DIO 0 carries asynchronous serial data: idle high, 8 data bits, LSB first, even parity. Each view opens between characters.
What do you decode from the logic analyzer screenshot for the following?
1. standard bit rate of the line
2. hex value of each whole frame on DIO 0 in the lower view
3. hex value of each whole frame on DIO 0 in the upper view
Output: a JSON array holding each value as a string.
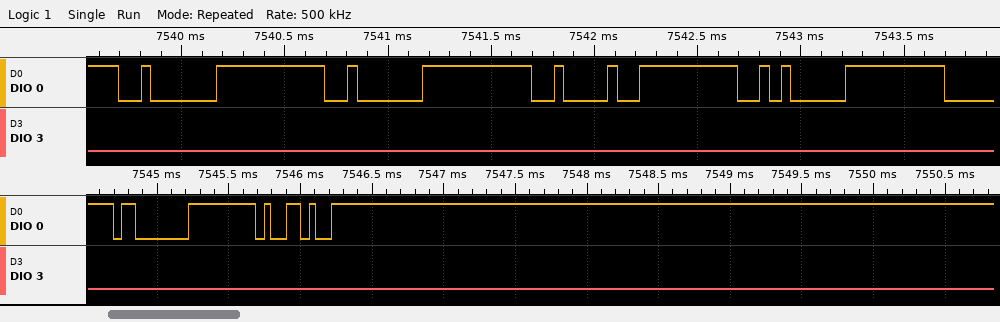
["19200 baud", "03, 59", "02, 02, 42, 0A"]
